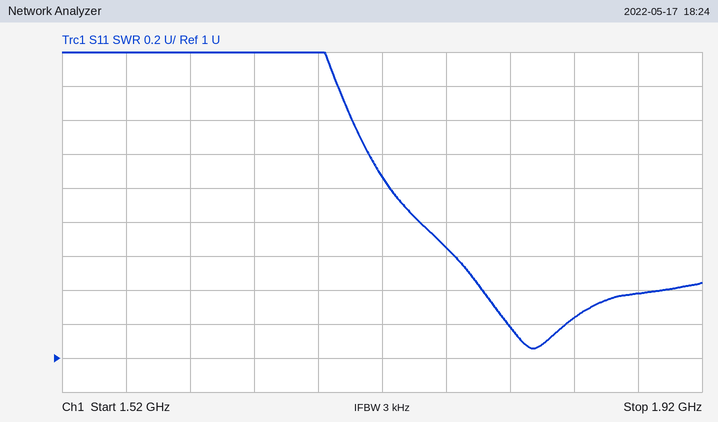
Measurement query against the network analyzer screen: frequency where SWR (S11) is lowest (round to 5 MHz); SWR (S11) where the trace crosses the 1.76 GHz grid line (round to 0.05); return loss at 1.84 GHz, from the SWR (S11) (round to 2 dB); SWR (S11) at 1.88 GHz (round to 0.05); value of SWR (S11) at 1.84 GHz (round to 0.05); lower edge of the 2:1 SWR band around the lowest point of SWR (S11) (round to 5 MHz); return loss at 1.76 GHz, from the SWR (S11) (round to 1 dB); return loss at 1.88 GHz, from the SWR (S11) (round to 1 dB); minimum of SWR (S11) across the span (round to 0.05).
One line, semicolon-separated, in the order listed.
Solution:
1.815 GHz; 1.65; 20 dB; 1.40; 1.25; 1.725 GHz; 12 dB; 16 dB; 1.05
